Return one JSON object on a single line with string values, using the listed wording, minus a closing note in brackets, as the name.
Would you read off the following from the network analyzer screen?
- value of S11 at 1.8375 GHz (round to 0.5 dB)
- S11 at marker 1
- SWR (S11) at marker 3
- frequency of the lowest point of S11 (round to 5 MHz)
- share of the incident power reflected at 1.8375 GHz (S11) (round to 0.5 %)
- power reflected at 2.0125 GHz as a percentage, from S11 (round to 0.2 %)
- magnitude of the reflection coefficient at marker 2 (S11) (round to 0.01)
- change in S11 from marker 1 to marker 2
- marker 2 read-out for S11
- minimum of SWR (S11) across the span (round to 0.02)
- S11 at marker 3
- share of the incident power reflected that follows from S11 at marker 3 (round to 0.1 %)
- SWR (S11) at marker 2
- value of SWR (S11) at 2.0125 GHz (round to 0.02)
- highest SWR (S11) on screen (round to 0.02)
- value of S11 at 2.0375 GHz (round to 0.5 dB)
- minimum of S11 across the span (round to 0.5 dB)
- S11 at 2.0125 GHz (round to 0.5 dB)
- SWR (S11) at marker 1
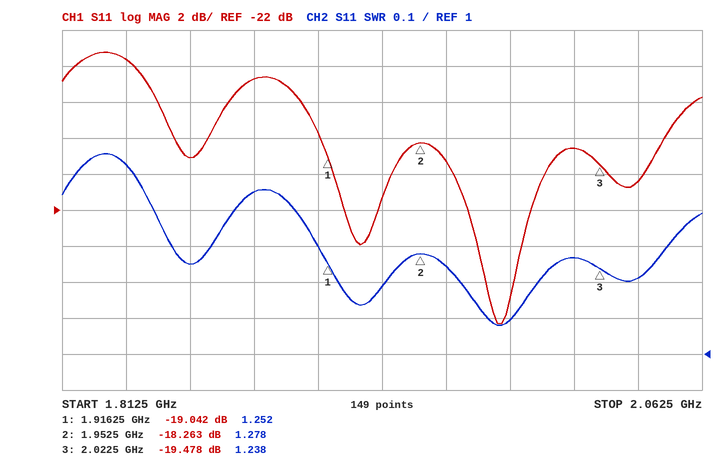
{"value of S11 at 1.8375 GHz": "-13.5 dB", "S11 at marker 1": "-19.042 dB", "SWR (S11) at marker 3": "1.238", "frequency of the lowest point of S11": "1.985 GHz", "share of the incident power reflected at 1.8375 GHz (S11)": "4.5 %", "power reflected at 2.0125 GHz as a percentage, from S11": "1.4 %", "magnitude of the reflection coefficient at marker 2 (S11)": "0.12", "change in S11 from marker 1 to marker 2": "0.779 dB", "marker 2 read-out for S11": "-18.263 dB", "minimum of SWR (S11) across the span": "1.08", "S11 at marker 3": "-19.478 dB", "share of the incident power reflected that follows from S11 at marker 3": "1.1 %", "SWR (S11) at marker 2": "1.278", "value of SWR (S11) at 2.0125 GHz": "1.26", "highest SWR (S11) on screen": "1.56", "value of S11 at 2.0375 GHz": "-20.5 dB", "minimum of S11 across the span": "-28.5 dB", "S11 at 2.0125 GHz": "-18.5 dB", "SWR (S11) at marker 1": "1.252"}
